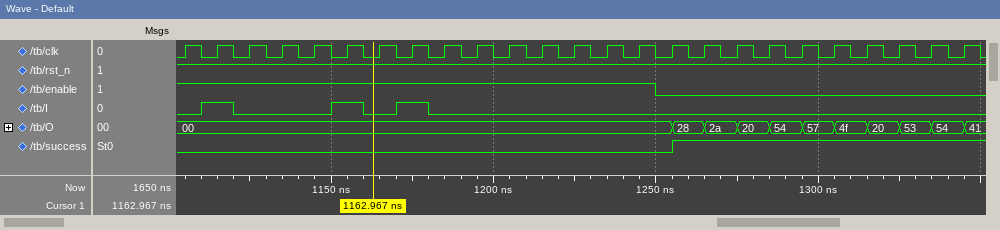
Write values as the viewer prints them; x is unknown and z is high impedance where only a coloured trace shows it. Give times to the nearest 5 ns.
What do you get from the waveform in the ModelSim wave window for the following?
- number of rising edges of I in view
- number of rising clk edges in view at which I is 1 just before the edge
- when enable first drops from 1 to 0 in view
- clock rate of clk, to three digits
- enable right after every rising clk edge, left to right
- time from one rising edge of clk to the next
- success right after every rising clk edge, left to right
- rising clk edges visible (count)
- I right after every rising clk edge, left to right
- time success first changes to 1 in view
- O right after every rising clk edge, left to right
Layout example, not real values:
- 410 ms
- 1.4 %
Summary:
- 3
- 3
- 1250 ns
- 100 MHz
- 1 1 1 1 1 1 1 1 1 1 1 1 1 1 1 0 0 0 0 0 0 0 0 0 0
- 10 ns
- 0 0 0 0 0 0 0 0 0 0 0 0 0 0 0 1 1 1 1 1 1 1 1 1 1
- 25
- 0 1 0 0 0 1 0 1 0 0 0 0 0 0 0 0 0 0 0 0 0 0 0 0 0
- 1255 ns
- 00, 00, 00, 00, 00, 00, 00, 00, 00, 00, 00, 00, 00, 00, 00, 28, 2a, 20, 54, 57, 4f, 20, 53, 54, 41
